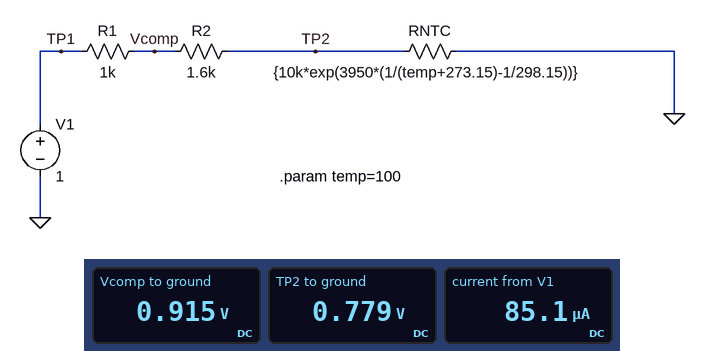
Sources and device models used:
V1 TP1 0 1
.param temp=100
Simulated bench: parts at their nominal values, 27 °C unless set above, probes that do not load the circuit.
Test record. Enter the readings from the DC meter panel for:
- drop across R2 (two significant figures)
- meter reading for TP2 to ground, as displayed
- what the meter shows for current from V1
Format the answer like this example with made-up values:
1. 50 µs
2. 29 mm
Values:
1. 140 mV
2. 0.779 V
3. 85.1 µA
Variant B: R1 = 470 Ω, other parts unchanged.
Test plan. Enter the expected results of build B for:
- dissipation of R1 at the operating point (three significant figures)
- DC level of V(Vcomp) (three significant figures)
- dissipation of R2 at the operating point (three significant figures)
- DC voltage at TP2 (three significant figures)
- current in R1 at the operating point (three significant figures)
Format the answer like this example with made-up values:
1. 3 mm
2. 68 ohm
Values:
1. 3.73 µW
2. 958 mV
3. 12.7 µW
4. 816 mV
5. 89.1 µA
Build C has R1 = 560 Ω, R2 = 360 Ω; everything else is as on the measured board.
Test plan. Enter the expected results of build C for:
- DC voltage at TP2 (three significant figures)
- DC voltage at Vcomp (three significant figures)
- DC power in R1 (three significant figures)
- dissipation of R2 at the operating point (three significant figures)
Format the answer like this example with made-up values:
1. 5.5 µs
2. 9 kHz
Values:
1. 909 mV
2. 944 mV
3. 5.52 µW
4. 3.55 µW
